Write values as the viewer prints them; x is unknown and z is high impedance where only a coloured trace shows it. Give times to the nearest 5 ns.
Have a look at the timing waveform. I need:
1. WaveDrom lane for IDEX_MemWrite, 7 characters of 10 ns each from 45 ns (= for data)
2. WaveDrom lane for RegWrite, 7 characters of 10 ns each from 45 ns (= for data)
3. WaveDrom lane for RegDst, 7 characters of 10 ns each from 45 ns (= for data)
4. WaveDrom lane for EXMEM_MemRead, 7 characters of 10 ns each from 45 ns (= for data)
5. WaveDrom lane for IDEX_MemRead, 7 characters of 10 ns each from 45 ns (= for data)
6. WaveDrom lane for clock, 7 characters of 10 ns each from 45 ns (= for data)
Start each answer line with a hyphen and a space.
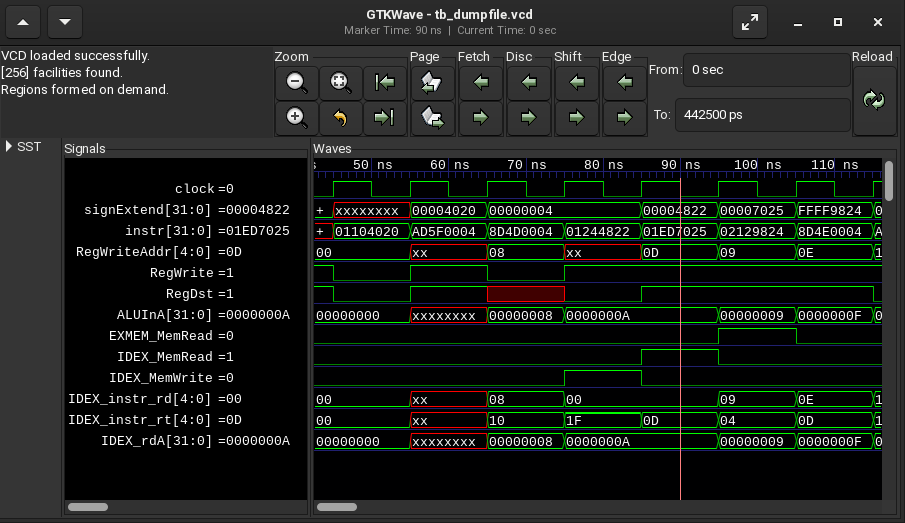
- {name: 'IDEX_MemWrite', wave: '0..10..'}
- {name: 'RegWrite', wave: '0101...'}
- {name: 'RegDst', wave: '01x01..'}
- {name: 'EXMEM_MemRead', wave: '0....10'}
- {name: 'IDEX_MemRead', wave: '0...10.'}
- {name: 'clock', wave: 'p......'}
